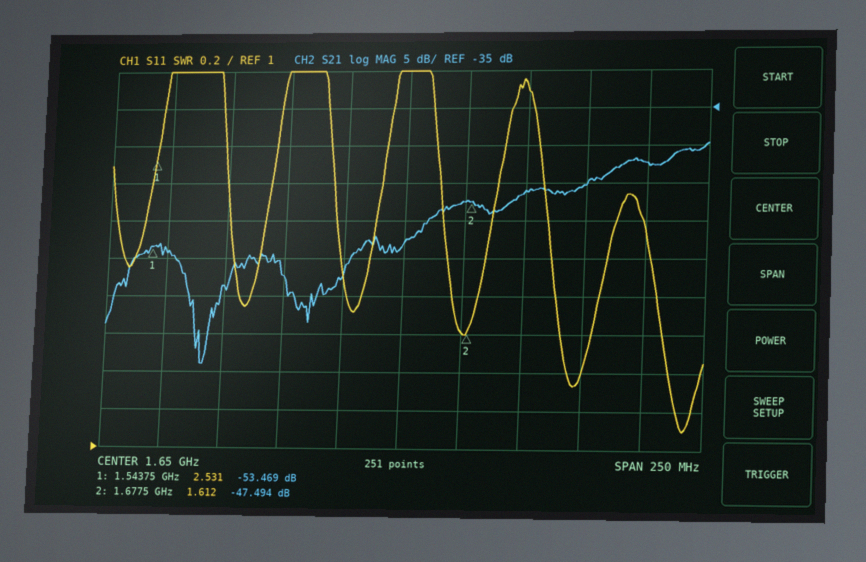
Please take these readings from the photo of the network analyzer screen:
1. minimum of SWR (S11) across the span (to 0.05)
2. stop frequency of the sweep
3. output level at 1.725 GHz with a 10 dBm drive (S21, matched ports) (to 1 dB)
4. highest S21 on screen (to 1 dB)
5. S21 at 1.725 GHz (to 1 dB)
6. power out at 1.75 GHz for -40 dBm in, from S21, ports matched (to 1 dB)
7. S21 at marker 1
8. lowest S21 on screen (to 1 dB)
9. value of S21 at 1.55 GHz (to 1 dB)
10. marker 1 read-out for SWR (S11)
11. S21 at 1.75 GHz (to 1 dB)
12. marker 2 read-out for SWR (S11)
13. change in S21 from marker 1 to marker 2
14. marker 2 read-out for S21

1.10
1.775 GHz
-35 dBm
-40 dB
-45 dB
-82 dBm
-53.469 dB
-69 dB
-54 dB
2.531
-42 dB
1.612
5.975 dB
-47.494 dB
